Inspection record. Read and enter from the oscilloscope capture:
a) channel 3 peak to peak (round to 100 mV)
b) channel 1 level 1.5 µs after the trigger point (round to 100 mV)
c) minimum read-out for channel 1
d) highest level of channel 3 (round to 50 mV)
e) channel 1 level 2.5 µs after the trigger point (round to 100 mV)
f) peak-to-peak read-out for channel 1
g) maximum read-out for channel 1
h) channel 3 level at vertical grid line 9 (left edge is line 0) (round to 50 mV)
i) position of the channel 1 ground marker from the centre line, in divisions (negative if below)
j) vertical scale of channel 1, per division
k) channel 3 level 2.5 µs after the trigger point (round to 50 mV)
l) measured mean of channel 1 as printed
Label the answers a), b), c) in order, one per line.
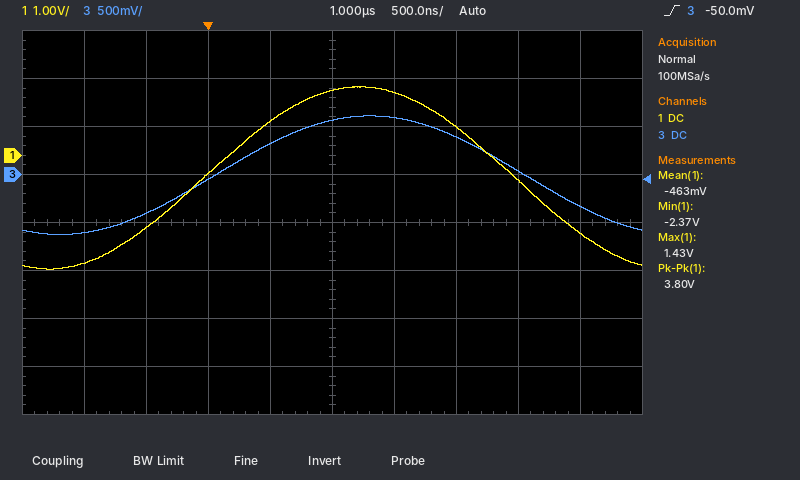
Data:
a) 1.20 V
b) 1.3 V
c) -2.37 V
d) 600 mV
e) -500 mV
f) 3.80 V
g) 1.43 V
h) -350 mV
i) +1.4 div
j) 1 V
k) 50 mV
l) -463 mV
